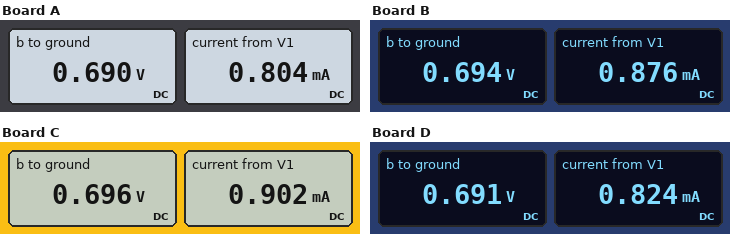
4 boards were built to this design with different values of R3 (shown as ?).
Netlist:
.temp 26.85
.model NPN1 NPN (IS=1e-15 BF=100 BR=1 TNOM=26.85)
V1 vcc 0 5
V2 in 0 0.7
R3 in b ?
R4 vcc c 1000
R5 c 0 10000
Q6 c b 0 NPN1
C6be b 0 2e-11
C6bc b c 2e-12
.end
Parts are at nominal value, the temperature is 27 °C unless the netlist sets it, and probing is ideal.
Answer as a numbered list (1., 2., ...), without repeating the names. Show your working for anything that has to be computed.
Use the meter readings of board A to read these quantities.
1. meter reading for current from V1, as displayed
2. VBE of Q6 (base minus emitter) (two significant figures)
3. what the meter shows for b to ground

1. 0.804 mA
2. 690 mV = 690 mV
3. 0.690 V
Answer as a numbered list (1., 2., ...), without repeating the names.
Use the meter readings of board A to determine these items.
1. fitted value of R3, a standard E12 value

1. 2.7 kΩ
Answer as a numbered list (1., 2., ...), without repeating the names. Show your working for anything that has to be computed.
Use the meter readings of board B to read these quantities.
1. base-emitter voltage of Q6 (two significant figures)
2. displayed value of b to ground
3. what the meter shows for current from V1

1. 694 mV = 690 mV
2. 0.694 V
3. 0.876 mA
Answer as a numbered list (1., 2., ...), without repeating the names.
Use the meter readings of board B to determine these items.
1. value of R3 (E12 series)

1. 1.2 kΩ
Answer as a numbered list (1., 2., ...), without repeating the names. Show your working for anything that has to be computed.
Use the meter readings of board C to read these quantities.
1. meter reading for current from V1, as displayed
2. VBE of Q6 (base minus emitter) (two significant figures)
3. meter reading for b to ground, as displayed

1. 0.902 mA
2. 696 mV = 700 mV
3. 0.696 V
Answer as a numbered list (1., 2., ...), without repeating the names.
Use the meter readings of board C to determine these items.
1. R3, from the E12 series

1. 820 Ω
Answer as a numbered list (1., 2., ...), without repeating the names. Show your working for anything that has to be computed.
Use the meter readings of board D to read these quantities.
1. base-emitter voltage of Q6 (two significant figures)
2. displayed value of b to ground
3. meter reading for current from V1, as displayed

1. 691 mV = 690 mV
2. 0.691 V
3. 0.824 mA
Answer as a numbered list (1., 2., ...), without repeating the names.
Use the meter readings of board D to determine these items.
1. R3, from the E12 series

1. 2.2 kΩ
